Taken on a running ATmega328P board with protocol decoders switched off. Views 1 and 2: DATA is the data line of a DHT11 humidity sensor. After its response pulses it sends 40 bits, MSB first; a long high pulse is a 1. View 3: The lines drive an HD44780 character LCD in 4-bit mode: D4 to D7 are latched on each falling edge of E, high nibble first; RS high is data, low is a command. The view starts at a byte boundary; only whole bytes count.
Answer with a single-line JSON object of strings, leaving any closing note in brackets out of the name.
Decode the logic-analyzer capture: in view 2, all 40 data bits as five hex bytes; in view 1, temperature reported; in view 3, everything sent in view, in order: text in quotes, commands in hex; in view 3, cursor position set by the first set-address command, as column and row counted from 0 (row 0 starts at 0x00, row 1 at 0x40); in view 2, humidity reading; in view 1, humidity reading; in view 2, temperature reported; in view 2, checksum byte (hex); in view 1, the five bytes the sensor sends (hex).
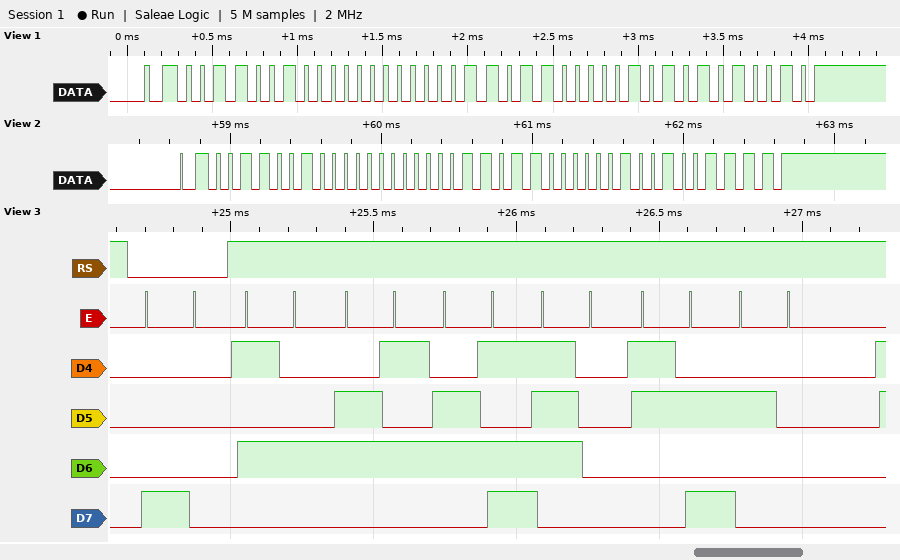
{"in view 2, all 40 data bits as five hex bytes": "32 00 1B 02 4F", "in view 1, temperature reported": "27.5 °C", "in view 3, everything sent in view, in order: text in quotes, commands in hex": "0x80 \"Temp: \"", "in view 3, cursor position set by the first set-address command, as column and row counted from 0": "column 0, row 0", "in view 2, humidity reading": "50 %", "in view 1, humidity reading": "50 %", "in view 2, temperature reported": "27.2 °C", "in view 2, checksum byte": "0x4F", "in view 1, the five bytes the sensor sends": "32 00 1B 05 52"}
